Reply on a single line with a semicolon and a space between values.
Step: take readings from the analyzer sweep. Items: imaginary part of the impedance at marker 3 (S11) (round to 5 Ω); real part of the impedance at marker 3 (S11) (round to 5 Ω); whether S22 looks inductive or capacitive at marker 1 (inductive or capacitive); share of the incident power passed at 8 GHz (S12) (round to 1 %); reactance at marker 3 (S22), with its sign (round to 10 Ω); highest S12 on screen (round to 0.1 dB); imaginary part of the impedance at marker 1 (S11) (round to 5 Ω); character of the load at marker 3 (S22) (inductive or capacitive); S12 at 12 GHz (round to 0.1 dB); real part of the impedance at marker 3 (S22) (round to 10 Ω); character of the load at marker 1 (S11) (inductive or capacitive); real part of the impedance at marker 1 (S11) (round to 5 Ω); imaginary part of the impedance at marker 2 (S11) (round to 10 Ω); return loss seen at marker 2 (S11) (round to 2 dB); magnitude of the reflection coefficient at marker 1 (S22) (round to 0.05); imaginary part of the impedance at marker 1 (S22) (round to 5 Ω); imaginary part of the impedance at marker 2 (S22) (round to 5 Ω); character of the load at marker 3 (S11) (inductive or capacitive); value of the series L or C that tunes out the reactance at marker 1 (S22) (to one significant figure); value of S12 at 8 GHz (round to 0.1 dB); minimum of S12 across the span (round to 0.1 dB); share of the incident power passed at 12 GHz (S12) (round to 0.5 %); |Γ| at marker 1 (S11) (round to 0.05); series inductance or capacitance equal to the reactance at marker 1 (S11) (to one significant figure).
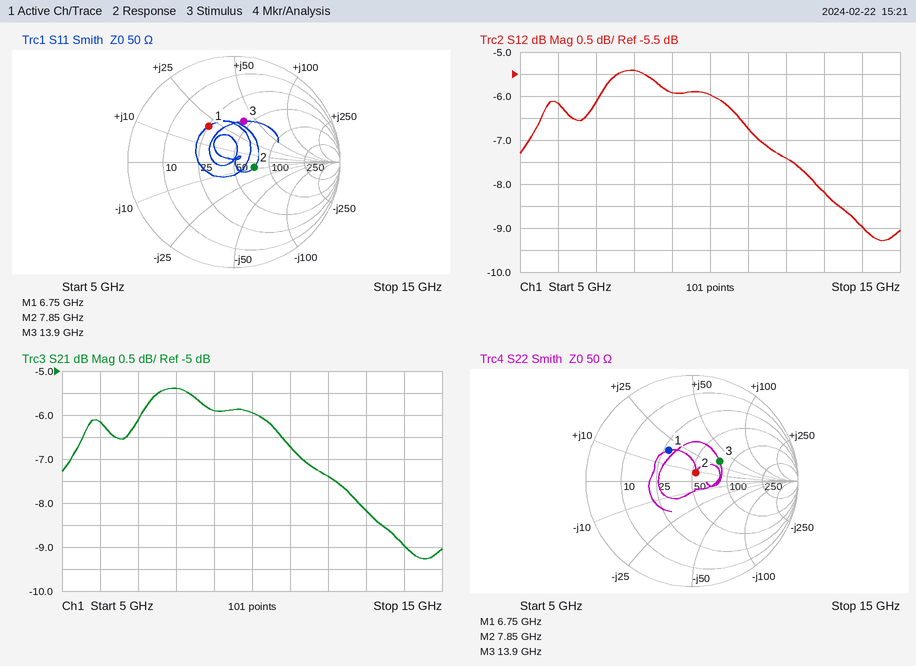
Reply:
+40 Ω; 45 Ω; inductive; 29 %; +30 Ω; -5.4 dB; +20 Ω; inductive; -7.4 dB; 80 Ω; inductive; 25 Ω; -10 Ω; 14 dB; 0.35; +20 Ω; +10 Ω; inductive; 1 pF; -5.4 dB; -9.3 dB; 18.0 %; 0.40; 500 pH
